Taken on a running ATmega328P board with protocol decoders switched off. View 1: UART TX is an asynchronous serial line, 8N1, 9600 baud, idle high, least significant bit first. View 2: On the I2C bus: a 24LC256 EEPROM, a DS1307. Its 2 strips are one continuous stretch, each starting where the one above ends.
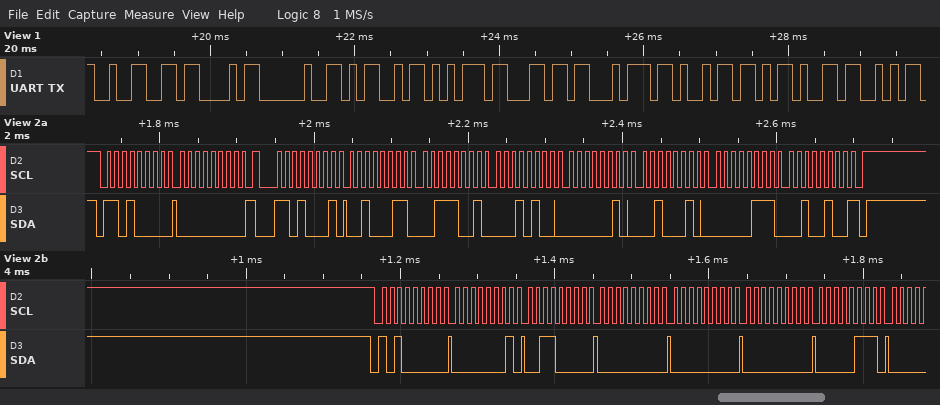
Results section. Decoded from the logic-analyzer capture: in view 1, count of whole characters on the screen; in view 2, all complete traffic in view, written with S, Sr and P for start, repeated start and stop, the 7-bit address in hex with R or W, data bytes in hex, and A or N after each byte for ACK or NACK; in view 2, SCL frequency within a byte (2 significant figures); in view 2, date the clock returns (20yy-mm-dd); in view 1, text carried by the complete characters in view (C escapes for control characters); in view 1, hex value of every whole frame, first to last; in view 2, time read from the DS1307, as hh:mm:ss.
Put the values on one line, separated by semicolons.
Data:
10; S 68W A 00 A Sr 68R A 23 A 39 A 14 A 02 A 22 A 07 A 24 N P S 50W A 01 A 30 A 00 A 00 A 00 A 07 A; 100 kHz; 2024-07-22; "2C Multi-S"; 32 43 20 4D 75 6C 74 69 2D 53; 14:39:23
